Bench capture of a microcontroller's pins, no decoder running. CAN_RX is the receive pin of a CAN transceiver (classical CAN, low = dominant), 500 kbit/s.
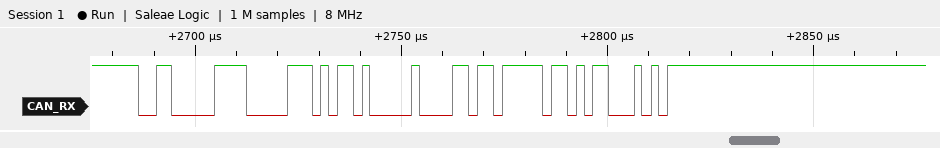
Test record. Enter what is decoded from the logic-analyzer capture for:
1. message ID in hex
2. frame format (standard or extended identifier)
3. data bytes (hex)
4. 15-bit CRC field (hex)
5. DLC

0x307
standard
5A 00 DB
0x7D62
3
